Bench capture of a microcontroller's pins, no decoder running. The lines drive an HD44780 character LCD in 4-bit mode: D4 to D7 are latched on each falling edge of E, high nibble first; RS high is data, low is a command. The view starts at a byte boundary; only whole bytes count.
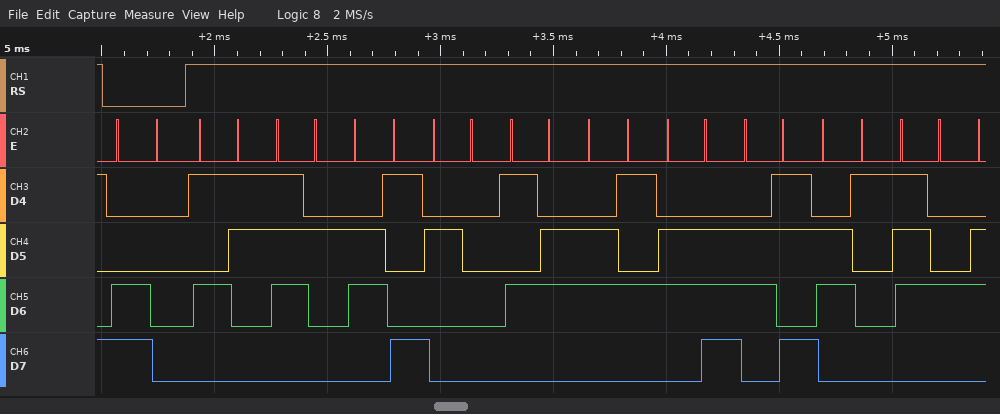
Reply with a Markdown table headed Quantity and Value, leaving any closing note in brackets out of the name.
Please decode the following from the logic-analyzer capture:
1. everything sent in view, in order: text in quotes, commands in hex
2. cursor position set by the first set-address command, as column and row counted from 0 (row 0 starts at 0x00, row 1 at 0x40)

| Quantity | Value |
|---|---|
| everything sent in view, in order: text in quotes, commands in hex | 0xC0 "Sri Venkat" |
| cursor position set by the first set-address command, as column and row counted from 0 | column 0, row 1 |
